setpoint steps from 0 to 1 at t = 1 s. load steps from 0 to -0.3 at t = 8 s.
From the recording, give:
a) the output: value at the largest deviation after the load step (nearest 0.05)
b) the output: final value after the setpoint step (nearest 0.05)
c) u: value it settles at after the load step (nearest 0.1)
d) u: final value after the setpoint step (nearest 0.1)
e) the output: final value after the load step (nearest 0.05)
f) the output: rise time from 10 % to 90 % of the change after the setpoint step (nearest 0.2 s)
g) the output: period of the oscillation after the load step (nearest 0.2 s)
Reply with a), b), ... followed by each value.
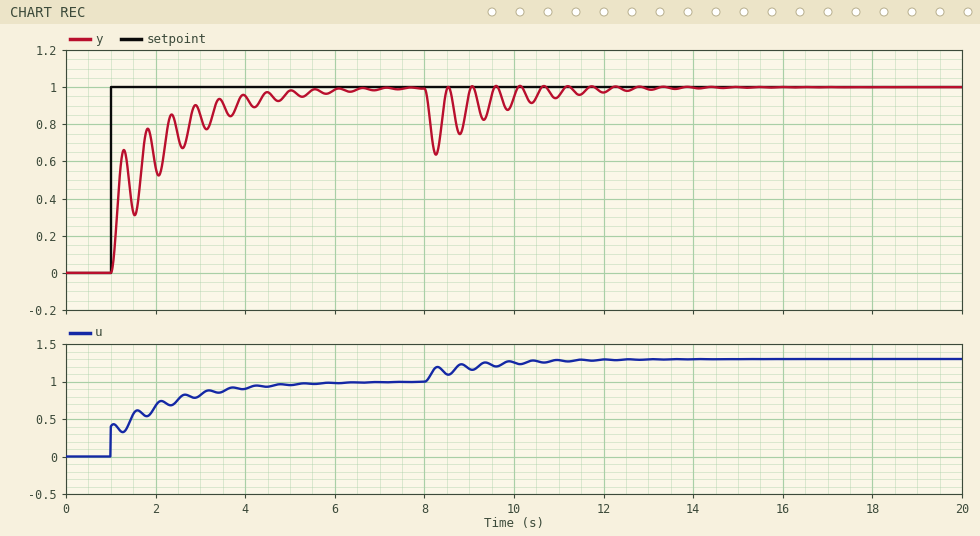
a) 0.65
b) 1.00
c) 1.3
d) 1.0
e) 1.00
f) 1.8 s
g) 0.6 s
